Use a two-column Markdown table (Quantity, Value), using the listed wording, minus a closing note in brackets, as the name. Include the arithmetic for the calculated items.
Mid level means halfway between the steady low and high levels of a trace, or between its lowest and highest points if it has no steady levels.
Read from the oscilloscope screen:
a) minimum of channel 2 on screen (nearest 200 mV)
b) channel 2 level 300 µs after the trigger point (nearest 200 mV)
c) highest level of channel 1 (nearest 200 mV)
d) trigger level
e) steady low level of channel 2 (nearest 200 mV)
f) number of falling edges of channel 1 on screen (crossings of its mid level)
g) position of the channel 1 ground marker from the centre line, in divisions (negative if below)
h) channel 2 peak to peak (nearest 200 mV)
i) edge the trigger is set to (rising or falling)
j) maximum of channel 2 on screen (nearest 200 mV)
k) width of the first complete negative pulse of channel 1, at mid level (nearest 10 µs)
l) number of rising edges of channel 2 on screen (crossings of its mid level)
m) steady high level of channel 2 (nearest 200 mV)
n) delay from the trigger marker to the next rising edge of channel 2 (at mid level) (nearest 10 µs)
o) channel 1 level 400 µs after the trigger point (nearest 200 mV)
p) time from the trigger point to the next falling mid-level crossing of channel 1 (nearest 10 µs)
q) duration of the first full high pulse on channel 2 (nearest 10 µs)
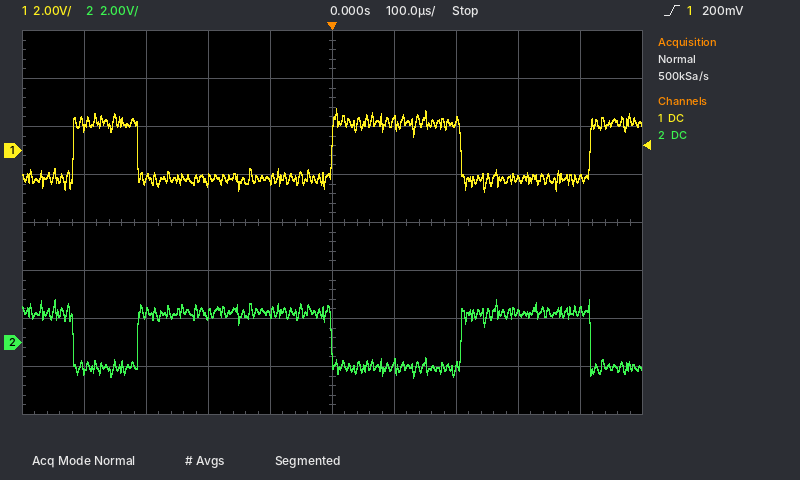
| Quantity | Value |
|---|---|
| minimum of channel 2 on screen | -1.4 V |
| channel 2 level 300 µs after the trigger point | 1.2 V |
| highest level of channel 1 | 1.8 V |
| trigger level | 200 mV |
| steady low level of channel 2 | -1.0 V |
| number of falling edges of channel 1 on screen | 2 |
| position of the channel 1 ground marker from the centre line, in divisions | +1.5 div |
| channel 2 peak to peak | 1.8 V − (-1.4 V) = 3.2 V |
| edge the trigger is set to | rising |
| maximum of channel 2 on screen | 1.8 V |
| width of the first complete negative pulse of channel 1, at mid level | 310 µs |
| number of rising edges of channel 2 on screen | 2 |
| steady high level of channel 2 | 1.2 V |
| delay from the trigger marker to the next rising edge of channel 2 (at mid level) | 210 µs |
| channel 1 level 400 µs after the trigger point | -1.2 V |
| time from the trigger point to the next falling mid-level crossing of channel 1 | 210 µs |
| duration of the first full high pulse on channel 2 | 310 µs |
